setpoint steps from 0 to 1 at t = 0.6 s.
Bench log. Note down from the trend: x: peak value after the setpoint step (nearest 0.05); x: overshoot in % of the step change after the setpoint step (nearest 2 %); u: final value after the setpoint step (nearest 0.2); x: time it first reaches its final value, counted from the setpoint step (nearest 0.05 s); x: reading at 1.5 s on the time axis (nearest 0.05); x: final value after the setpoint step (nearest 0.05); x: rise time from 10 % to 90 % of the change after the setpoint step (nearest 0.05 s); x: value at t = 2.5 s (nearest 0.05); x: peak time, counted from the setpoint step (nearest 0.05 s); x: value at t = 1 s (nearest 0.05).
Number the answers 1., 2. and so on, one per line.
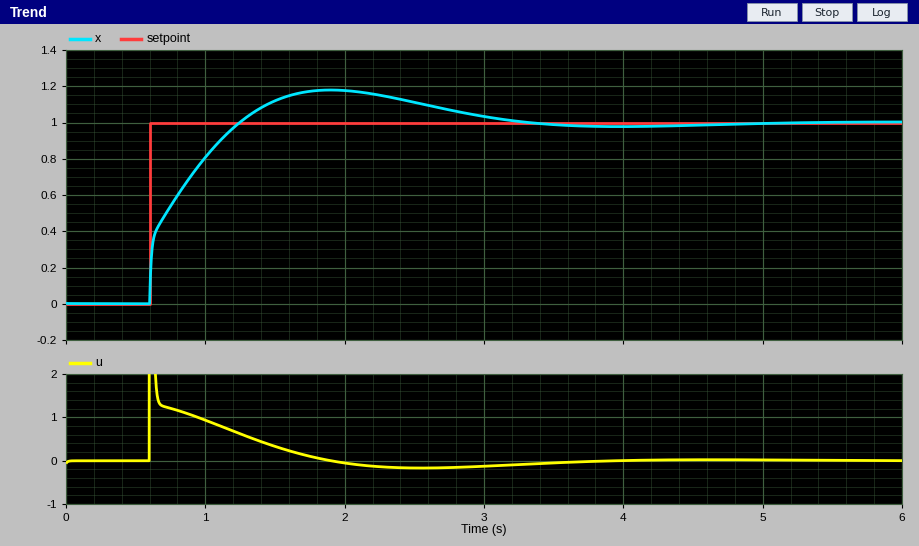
1. 1.20
2. 18 %
3. 0.0
4. 0.65 s
5. 1.10
6. 1.00
7. 0.50 s
8. 1.10
9. 1.30 s
10. 0.80
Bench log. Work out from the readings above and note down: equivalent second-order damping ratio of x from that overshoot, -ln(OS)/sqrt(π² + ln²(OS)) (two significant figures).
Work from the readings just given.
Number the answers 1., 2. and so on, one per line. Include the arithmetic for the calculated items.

1. ln(0.18) = -1.715; 1.715 / sqrt(9.870 + 2.941) = 0.48
